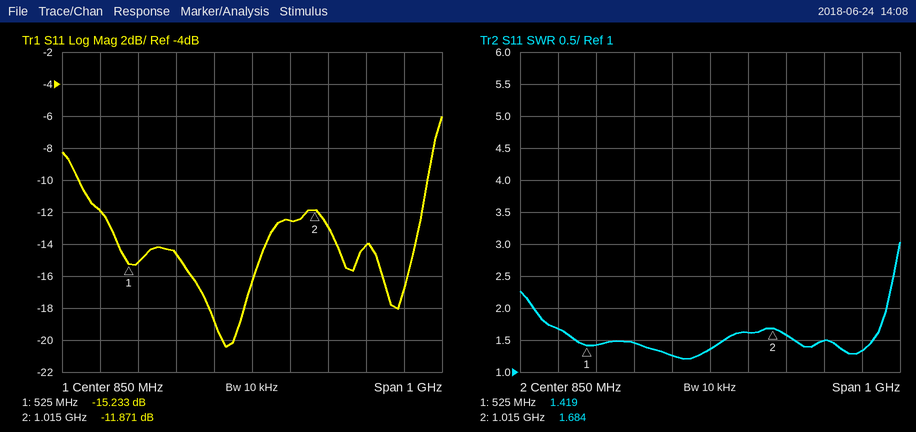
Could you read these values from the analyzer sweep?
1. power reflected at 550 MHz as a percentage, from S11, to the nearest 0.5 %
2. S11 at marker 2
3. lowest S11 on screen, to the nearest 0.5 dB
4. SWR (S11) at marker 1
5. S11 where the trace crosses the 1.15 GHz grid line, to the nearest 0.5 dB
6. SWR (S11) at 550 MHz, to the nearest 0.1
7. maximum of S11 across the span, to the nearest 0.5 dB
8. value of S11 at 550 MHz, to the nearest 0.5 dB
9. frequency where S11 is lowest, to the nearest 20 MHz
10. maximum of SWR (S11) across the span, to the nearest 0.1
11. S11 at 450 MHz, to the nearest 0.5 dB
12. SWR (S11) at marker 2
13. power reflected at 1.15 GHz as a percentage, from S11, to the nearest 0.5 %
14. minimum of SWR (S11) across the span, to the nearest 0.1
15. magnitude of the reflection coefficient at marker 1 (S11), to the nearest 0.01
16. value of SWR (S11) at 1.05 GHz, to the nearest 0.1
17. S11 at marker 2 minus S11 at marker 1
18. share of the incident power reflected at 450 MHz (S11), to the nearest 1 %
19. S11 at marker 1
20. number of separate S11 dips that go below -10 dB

3.0 %
-11.871 dB
-20.5 dB
1.419
-14.0 dB
1.4
-6.0 dB
-15.0 dB
780 MHz
3.0
-12.0 dB
1.684
4.0 %
1.2
0.17
1.6
3.362 dB
6 %
-15.233 dB
2
